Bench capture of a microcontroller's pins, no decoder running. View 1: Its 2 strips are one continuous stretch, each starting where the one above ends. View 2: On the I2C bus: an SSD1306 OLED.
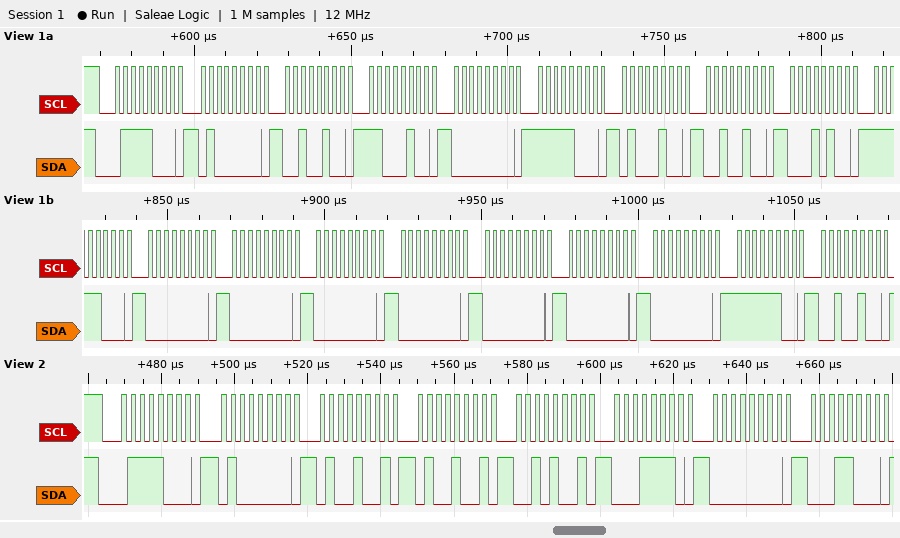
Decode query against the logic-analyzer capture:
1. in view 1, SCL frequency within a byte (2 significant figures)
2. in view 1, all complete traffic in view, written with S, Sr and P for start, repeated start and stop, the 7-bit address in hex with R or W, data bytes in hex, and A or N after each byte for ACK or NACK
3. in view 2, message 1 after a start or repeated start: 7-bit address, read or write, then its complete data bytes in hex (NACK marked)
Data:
400 kHz
S 3CW A 40 A 24 A C4 A 00 A F8 A 44 A 24 A 14 A F8 A 00 A 00 A 00 A 00 A 00 A 00 A 00 A FC A 24 A
0x3C write: 40 49 49 29 1E 00 18
